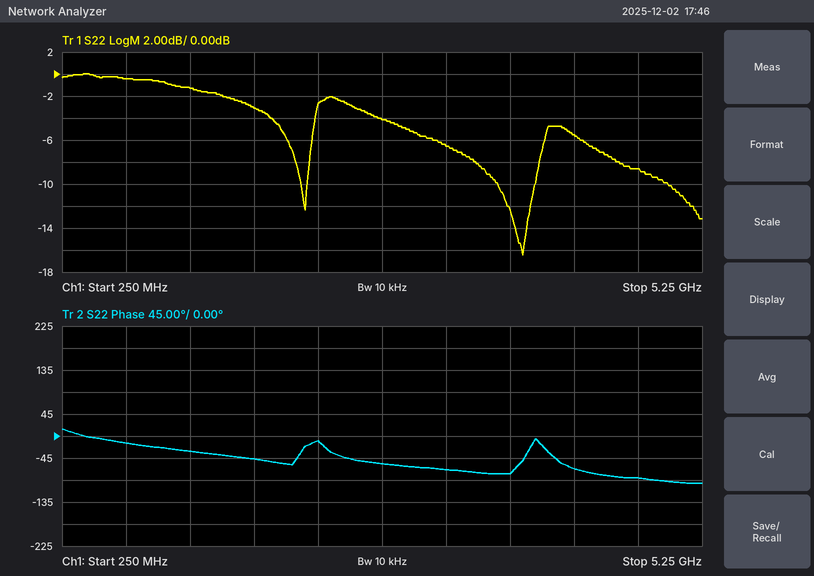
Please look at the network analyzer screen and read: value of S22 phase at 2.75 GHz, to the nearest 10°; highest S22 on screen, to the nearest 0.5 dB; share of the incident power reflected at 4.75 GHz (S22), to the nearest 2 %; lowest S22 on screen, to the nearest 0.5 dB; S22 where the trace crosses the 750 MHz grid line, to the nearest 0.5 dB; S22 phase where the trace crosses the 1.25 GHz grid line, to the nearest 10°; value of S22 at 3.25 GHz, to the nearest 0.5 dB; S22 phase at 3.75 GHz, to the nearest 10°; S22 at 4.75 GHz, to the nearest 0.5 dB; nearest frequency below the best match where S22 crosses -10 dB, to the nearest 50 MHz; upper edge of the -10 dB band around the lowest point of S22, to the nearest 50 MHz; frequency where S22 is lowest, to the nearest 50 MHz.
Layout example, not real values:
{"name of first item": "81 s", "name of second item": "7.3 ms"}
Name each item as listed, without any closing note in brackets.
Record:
{"value of S22 phase at 2.75 GHz, to the nearest 10°": "-60°", "highest S22 on screen, to the nearest 0.5 dB": "0.0 dB", "share of the incident power reflected at 4.75 GHz (S22), to the nearest 2 %": "14 %", "lowest S22 on screen, to the nearest 0.5 dB": "-16.5 dB", "S22 where the trace crosses the 750 MHz grid line, to the nearest 0.5 dB": "-0.5 dB", "S22 phase where the trace crosses the 1.25 GHz grid line, to the nearest 10°": "-30°", "value of S22 at 3.25 GHz, to the nearest 0.5 dB": "-6.5 dB", "S22 phase at 3.75 GHz, to the nearest 10°": "-80°", "S22 at 4.75 GHz, to the nearest 0.5 dB": "-8.5 dB", "nearest frequency below the best match where S22 crosses -10 dB, to the nearest 50 MHz": "3.65 GHz", "upper edge of the -10 dB band around the lowest point of S22, to the nearest 50 MHz": "3.95 GHz", "frequency where S22 is lowest, to the nearest 50 MHz": "3.85 GHz"}
